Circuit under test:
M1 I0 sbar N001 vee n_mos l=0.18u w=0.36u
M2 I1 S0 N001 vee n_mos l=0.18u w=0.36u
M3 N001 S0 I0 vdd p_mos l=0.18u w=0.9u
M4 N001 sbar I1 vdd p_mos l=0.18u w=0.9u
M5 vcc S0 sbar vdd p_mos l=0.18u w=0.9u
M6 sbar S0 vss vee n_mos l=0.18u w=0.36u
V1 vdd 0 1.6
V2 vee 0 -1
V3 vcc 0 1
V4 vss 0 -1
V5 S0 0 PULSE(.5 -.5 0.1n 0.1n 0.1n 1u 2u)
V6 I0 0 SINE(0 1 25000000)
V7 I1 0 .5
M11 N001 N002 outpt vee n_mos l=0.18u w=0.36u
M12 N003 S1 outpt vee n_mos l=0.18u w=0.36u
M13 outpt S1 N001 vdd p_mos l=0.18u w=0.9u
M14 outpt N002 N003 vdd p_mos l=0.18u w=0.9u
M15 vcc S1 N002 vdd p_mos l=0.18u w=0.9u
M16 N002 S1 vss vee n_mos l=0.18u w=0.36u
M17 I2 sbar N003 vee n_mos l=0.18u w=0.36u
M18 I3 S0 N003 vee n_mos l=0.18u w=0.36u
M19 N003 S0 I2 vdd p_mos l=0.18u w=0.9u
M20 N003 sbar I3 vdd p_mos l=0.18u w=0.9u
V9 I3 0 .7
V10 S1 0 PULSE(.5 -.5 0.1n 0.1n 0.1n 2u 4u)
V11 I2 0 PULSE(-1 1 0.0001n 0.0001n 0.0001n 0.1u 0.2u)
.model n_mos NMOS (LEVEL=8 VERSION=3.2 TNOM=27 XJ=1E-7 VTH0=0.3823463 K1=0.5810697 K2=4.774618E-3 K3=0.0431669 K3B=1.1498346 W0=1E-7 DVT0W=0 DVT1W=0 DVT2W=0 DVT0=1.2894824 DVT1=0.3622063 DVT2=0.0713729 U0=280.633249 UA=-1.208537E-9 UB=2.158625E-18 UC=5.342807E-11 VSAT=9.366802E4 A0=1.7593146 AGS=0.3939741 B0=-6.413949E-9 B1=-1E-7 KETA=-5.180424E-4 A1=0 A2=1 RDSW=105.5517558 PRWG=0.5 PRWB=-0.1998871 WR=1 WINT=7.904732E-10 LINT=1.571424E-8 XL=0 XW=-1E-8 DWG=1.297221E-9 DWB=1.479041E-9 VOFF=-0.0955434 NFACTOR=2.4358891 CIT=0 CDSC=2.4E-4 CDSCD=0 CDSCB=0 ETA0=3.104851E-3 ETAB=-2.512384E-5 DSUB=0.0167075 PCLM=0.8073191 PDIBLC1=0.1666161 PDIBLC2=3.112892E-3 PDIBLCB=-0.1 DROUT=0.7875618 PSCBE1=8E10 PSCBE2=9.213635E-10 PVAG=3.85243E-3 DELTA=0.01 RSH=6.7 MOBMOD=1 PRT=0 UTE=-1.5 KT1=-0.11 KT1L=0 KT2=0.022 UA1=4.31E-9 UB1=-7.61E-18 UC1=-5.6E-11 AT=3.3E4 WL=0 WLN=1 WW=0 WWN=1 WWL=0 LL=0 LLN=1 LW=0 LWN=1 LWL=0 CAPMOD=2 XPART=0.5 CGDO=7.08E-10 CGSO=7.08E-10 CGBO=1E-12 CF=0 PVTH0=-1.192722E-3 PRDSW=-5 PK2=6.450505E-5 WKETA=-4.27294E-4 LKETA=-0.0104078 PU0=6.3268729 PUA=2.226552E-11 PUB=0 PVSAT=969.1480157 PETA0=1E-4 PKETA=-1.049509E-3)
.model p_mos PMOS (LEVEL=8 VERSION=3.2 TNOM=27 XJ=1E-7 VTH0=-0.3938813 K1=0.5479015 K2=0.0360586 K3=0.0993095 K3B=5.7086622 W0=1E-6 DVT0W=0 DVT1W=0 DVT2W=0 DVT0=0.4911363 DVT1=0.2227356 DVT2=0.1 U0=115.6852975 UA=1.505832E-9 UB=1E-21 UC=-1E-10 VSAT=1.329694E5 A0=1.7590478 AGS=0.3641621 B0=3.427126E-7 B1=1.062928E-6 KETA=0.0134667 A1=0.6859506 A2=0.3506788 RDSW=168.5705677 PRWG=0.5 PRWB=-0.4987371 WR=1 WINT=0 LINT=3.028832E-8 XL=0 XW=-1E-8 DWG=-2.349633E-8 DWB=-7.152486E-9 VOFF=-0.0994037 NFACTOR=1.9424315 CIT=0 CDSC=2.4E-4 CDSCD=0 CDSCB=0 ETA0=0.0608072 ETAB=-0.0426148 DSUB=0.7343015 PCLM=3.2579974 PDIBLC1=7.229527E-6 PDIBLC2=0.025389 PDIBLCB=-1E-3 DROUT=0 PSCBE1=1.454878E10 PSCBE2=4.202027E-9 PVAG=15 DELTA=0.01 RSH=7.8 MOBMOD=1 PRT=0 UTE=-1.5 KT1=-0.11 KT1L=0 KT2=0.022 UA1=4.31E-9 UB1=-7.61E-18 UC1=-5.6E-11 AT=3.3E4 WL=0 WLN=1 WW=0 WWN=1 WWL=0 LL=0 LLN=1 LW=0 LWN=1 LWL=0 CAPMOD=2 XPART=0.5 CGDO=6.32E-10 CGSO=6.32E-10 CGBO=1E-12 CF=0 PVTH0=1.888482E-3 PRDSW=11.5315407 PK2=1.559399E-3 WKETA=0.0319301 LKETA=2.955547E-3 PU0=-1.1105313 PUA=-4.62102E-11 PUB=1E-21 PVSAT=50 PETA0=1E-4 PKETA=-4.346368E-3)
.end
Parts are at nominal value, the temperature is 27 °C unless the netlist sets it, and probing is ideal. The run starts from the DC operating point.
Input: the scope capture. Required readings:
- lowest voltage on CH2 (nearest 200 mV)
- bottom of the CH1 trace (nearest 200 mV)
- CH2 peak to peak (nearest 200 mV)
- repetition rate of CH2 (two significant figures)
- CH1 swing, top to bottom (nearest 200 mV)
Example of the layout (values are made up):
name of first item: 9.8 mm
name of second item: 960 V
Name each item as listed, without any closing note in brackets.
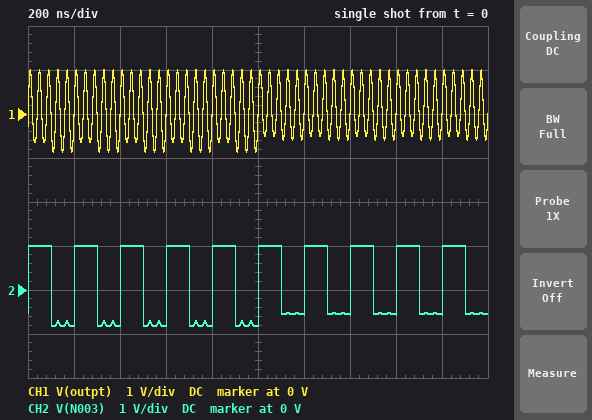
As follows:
lowest voltage on CH2: -800 mV
bottom of the CH1 trace: -800 mV
CH2 peak to peak: 1.8 V
repetition rate of CH2: 5.0 MHz
CH1 swing, top to bottom: 1.8 V
